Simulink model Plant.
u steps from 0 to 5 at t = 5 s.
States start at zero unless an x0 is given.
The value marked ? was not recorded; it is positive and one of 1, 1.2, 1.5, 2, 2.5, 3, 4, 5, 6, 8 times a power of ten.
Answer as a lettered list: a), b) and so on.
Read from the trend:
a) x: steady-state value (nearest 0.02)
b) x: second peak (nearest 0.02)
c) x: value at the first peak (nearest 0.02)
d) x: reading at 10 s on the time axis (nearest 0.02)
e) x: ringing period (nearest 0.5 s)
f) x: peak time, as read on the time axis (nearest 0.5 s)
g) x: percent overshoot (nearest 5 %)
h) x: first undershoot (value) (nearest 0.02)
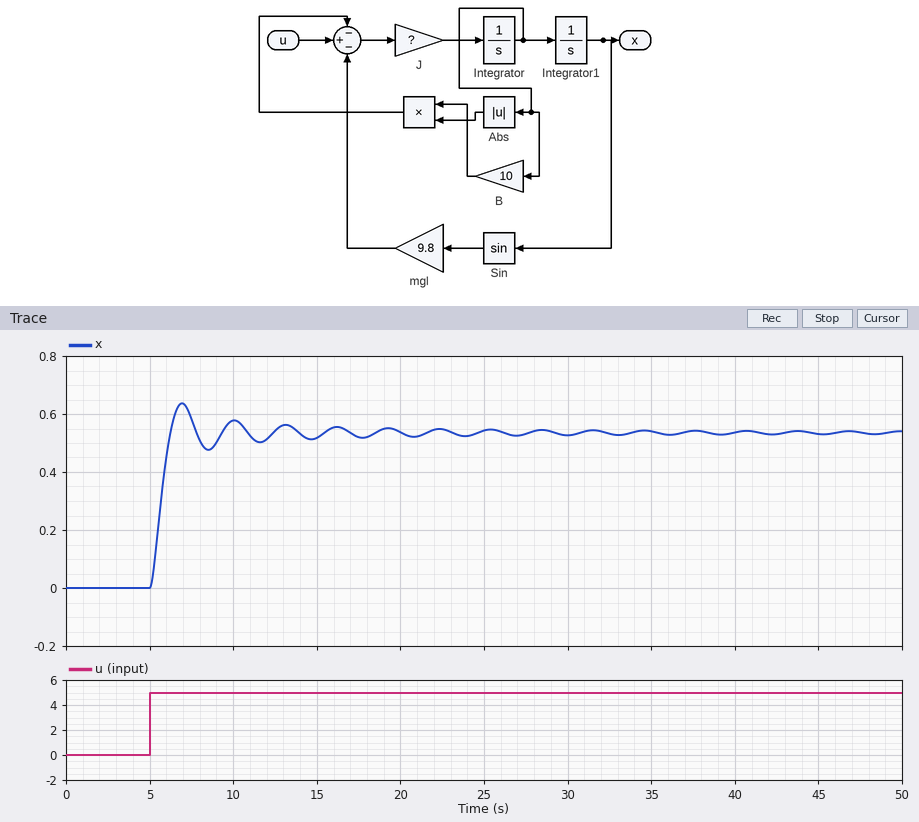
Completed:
a) 0.54
b) 0.58
c) 0.64
d) 0.58
e) 3.0 s
f) 7.0 s
g) 20 %
h) 0.48
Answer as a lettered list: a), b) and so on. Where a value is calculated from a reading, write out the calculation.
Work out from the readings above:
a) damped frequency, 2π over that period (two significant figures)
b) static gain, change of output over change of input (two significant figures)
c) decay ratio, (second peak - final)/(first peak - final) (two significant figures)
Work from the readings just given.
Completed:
a) 2π / 3 = 2.1 rad/s
b) (0.54 - 0) / (5 - 0) = 0.11
c) (0.58 - 0.54) / (0.64 - 0.54) = 0.40
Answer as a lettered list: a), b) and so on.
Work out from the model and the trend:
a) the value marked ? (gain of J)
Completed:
a) 0.5
